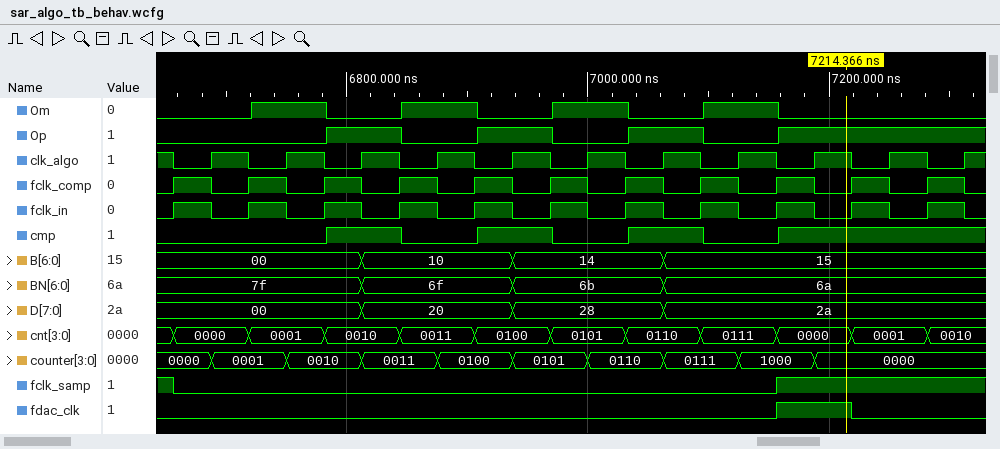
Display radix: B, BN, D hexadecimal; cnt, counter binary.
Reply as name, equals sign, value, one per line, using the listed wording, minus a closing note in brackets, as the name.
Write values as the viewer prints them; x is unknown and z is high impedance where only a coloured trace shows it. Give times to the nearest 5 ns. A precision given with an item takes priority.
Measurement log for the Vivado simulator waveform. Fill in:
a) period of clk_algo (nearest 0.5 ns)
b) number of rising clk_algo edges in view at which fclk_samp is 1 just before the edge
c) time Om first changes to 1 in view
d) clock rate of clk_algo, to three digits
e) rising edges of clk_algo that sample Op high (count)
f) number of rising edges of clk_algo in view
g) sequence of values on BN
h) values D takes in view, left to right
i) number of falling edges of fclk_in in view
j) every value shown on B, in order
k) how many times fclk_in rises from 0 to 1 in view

period of clk_algo = 62.5 ns
number of rising clk_algo edges in view at which fclk_samp is 1 just before the edge = 3
time Om first changes to 1 in view = 6720 ns
clock rate of clk_algo, to three digits = 16.0 MHz
rising edges of clk_algo that sample Op high = 6
number of rising edges of clk_algo in view = 11
sequence of values on BN = 7f, 6f, 6b, 6a
values D takes in view, left to right = 00, 20, 28, 2a
number of falling edges of fclk_in in view = 11
every value shown on B, in order = 00, 10, 14, 15
how many times fclk_in rises from 0 to 1 in view = 11
